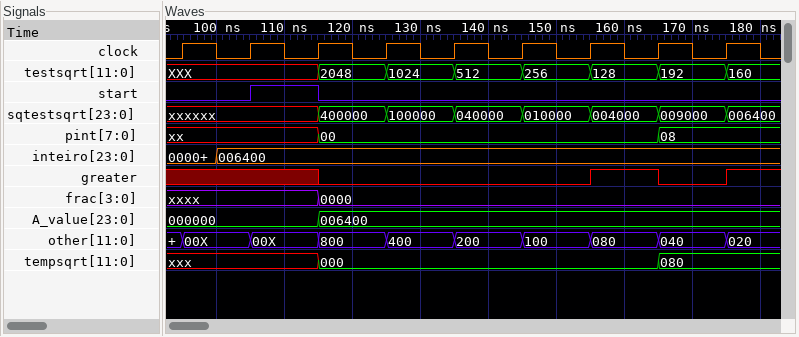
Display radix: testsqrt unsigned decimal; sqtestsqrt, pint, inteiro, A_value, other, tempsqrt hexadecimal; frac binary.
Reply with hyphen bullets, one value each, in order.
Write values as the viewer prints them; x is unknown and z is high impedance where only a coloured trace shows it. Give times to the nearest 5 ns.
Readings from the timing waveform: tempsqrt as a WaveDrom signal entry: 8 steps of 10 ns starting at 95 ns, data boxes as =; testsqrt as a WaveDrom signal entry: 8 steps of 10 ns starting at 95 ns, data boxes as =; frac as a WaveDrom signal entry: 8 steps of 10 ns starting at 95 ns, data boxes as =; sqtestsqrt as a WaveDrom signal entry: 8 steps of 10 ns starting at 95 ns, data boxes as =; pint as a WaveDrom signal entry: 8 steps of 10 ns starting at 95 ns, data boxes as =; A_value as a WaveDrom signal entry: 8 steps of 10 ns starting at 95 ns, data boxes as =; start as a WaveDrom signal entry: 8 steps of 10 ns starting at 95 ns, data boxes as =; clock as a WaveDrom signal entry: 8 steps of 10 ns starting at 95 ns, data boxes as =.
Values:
- {name: 'tempsqrt', wave: 'x.=....=', data: '000 080'}
- {name: 'testsqrt', wave: 'x.======', data: '2048 1024 512 256 128 192'}
- {name: 'frac', wave: 'x.=.....', data: '0000'}
- {name: 'sqtestsqrt', wave: 'x.======', data: '400000 100000 040000 010000 004000 009000'}
- {name: 'pint', wave: 'x.=....=', data: '00 08'}
- {name: 'A_value', wave: '=.=.....', data: '000000 006400'}
- {name: 'start', wave: '010.....'}
- {name: 'clock', wave: 'p.......'}
